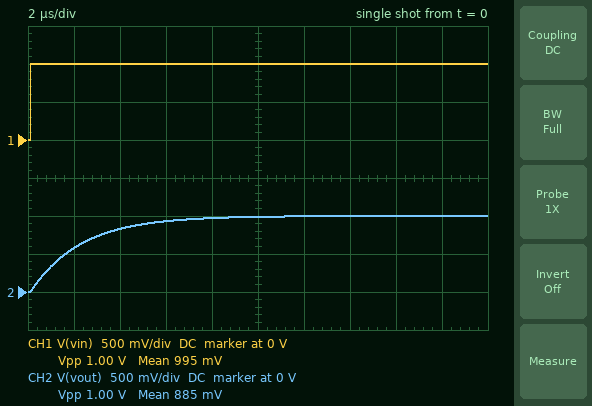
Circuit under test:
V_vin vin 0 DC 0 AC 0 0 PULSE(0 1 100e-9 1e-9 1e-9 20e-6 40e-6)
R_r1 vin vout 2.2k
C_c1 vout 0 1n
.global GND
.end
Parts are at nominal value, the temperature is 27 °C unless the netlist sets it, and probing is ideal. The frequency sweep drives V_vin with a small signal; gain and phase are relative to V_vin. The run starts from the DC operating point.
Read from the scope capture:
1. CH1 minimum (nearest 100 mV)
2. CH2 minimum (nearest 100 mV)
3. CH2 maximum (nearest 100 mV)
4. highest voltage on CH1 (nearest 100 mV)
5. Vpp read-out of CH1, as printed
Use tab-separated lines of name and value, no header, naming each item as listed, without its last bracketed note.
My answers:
CH1 minimum	0 V
CH2 minimum	0 V
CH2 maximum	1.0 V
highest voltage on CH1	1.0 V
Vpp read-out of CH1, as printed	1.00 V
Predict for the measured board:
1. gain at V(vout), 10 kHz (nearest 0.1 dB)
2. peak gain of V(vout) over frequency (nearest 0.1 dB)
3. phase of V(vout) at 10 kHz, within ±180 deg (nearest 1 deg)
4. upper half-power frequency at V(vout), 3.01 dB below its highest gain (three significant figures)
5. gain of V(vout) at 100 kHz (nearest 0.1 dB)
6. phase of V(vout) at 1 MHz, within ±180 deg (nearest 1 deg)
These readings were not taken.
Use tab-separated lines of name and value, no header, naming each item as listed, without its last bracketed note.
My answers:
gain at V(vout), 10 kHz	-0.1 dB
peak gain of V(vout) over frequency	0 dB
phase of V(vout) at 10 kHz, within ±180 deg	-8 deg
upper half-power frequency at V(vout), 3.01 dB below its highest gain	72.3 kHz
gain of V(vout) at 100 kHz	-4.6 dB
phase of V(vout) at 1 MHz, within ±180 deg	-86 deg
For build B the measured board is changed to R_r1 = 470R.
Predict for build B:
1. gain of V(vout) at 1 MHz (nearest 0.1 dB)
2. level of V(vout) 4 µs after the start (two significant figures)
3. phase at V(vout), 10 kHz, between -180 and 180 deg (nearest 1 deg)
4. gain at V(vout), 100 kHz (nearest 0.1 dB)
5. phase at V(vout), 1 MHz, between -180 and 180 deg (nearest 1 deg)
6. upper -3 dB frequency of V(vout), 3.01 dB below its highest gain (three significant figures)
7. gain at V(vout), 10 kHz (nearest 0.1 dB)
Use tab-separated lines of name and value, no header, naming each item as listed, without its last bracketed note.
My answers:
gain of V(vout) at 1 MHz	-9.9 dB
level of V(vout) 4 µs after the start	1.0 V
phase at V(vout), 10 kHz, between -180 and 180 deg	-2 deg
gain at V(vout), 100 kHz	-0.4 dB
phase at V(vout), 1 MHz, between -180 and 180 deg	-71 deg
upper -3 dB frequency of V(vout), 3.01 dB below its highest gain	339 kHz
gain at V(vout), 10 kHz	0 dB
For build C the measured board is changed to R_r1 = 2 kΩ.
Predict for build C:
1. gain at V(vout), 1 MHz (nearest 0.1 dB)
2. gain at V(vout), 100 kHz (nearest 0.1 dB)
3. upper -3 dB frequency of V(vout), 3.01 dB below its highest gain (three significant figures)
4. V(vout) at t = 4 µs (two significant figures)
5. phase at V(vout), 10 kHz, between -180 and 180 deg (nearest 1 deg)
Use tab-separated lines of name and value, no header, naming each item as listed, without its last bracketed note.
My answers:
gain at V(vout), 1 MHz	-22.0 dB
gain at V(vout), 100 kHz	-4.1 dB
upper -3 dB frequency of V(vout), 3.01 dB below its highest gain	79.6 kHz
V(vout) at t = 4 µs	860 mV
phase at V(vout), 10 kHz, between -180 and 180 deg	-7 deg
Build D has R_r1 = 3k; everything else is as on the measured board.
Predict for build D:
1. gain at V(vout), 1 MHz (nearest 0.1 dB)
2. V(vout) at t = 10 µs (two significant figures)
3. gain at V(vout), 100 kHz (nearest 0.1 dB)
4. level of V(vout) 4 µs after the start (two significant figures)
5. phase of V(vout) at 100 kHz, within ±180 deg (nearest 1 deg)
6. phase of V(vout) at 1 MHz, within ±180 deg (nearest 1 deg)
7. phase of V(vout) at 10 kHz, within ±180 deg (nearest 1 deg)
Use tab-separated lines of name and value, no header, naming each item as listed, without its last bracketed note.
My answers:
gain at V(vout), 1 MHz	-25.5 dB
V(vout) at t = 10 µs	960 mV
gain at V(vout), 100 kHz	-6.6 dB
level of V(vout) 4 µs after the start	730 mV
phase of V(vout) at 100 kHz, within ±180 deg	-62 deg
phase of V(vout) at 1 MHz, within ±180 deg	-87 deg
phase of V(vout) at 10 kHz, within ±180 deg	-11 deg
